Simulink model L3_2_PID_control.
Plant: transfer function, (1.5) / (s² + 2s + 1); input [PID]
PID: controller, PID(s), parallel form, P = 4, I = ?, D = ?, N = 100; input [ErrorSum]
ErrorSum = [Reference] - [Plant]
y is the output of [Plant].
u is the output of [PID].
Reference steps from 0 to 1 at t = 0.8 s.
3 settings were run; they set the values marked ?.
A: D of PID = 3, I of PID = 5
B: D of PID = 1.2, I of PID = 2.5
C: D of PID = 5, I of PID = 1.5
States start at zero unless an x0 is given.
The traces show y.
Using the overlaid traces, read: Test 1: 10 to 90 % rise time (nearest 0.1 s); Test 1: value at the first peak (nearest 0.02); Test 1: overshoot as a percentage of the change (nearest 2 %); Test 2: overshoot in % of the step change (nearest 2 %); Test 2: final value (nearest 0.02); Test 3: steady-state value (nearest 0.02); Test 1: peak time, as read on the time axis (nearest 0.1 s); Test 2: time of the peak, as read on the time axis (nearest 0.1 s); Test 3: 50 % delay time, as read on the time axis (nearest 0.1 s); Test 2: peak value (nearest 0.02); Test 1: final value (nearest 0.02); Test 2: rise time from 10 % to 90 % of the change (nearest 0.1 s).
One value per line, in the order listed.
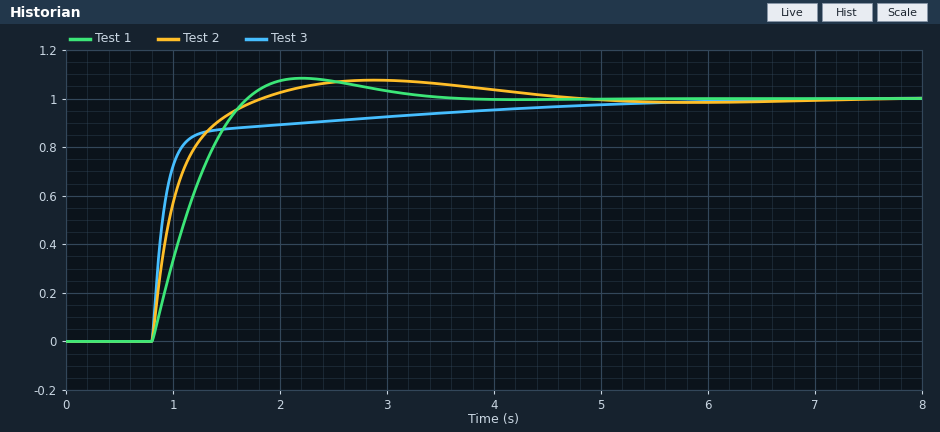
0.6 s
1.08
8 %
8 %
1.00
1.00
2.2 s
2.9 s
0.9 s
1.08
1.00
0.6 s
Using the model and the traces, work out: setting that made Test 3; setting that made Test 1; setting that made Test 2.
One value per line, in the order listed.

C
B
A
